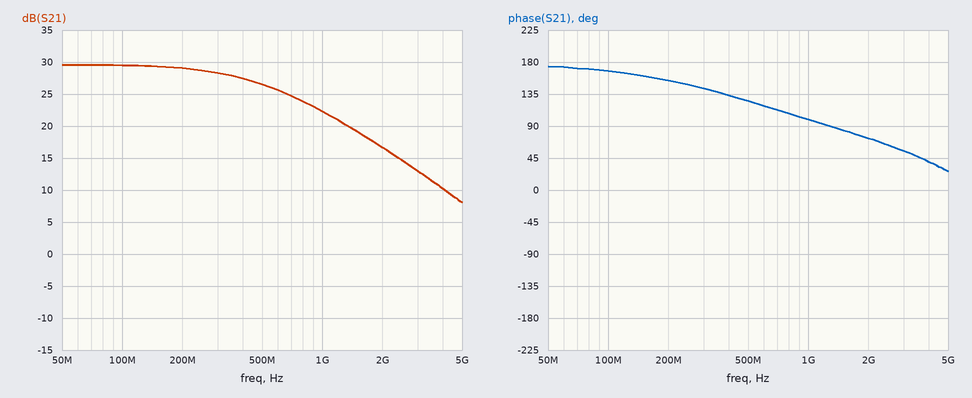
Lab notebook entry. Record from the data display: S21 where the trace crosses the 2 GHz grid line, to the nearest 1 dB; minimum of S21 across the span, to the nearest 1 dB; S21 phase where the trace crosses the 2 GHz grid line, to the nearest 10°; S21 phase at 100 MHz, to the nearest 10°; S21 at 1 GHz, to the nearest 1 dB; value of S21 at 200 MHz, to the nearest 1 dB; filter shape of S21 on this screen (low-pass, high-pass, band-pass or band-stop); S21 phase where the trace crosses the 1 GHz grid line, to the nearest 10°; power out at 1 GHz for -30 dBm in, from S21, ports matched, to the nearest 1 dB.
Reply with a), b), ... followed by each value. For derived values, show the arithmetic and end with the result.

a) 17 dB
b) 8 dB
c) 70°
d) 170°
e) 22 dB
f) 29 dB
g) low-pass
h) 100°
i) -30 dBm + (22 dB) = -8 dBm
